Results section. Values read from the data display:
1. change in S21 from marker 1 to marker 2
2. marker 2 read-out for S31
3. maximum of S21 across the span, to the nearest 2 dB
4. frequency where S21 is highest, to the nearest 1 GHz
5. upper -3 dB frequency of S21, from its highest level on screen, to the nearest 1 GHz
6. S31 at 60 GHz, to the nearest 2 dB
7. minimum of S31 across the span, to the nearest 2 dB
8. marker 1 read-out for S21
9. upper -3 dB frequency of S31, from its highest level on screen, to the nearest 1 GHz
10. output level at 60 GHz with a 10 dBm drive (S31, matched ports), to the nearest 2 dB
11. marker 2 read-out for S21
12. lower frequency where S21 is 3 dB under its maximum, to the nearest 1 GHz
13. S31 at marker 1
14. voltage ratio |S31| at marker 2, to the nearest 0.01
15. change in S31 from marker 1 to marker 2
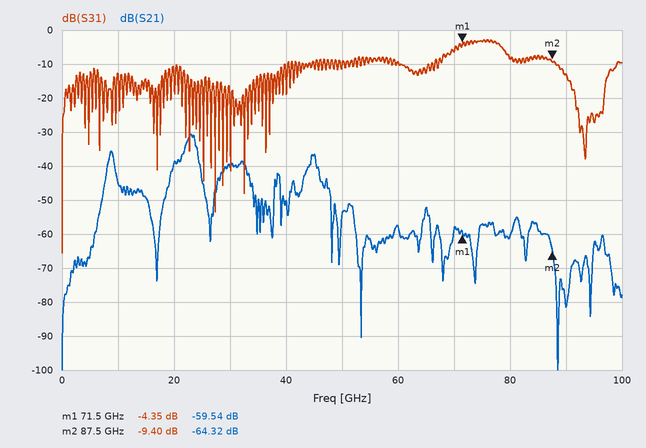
-4.78 dB
-9.40 dB
-30 dB
23 GHz
24 GHz
-10 dB
-66 dB
-59.54 dB
79 GHz
0 dBm
-64.32 dB
22 GHz
-4.35 dB
0.34
-5.05 dB
